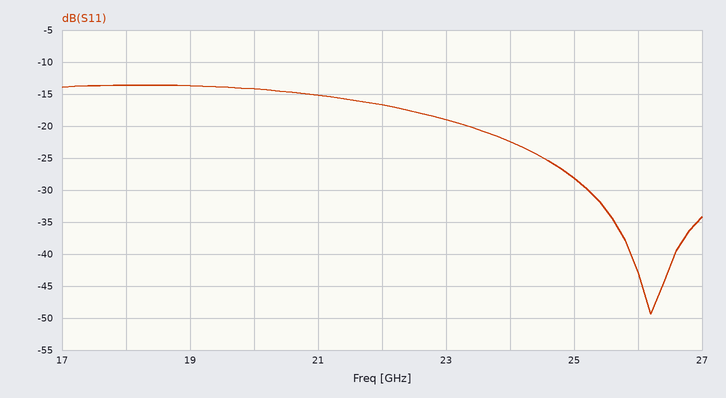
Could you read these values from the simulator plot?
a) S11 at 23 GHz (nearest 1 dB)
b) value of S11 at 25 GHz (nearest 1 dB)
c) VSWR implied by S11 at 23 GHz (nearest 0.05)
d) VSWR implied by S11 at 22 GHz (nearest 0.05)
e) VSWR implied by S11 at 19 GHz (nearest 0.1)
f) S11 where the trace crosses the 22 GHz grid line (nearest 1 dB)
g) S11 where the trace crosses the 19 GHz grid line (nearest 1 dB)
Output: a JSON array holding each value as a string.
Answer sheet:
["-19 dB", "-28 dB", "1.25", "1.35", "1.5", "-17 dB", "-14 dB"]
